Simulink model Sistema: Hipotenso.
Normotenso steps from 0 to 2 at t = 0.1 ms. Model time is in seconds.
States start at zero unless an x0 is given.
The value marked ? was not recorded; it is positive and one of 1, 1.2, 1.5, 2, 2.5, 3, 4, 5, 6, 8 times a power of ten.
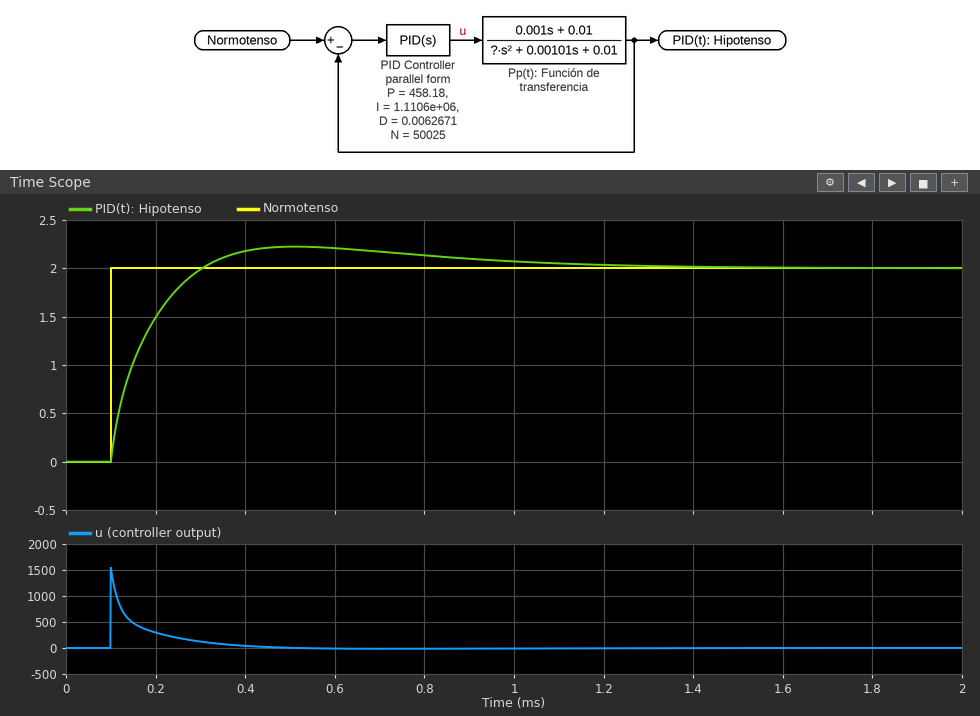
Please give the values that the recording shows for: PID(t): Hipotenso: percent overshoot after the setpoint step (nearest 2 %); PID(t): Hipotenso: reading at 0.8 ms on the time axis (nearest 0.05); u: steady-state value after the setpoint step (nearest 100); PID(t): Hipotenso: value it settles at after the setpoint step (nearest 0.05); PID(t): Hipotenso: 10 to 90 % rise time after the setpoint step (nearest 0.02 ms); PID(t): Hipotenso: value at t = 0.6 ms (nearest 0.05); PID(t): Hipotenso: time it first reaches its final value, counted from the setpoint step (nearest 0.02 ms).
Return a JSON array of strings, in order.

["12 %", "2.15", "0", "2.00", "0.14 ms", "2.20", "0.20 ms"]
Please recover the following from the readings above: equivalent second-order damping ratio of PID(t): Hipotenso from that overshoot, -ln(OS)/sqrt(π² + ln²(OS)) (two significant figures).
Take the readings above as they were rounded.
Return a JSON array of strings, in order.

["0.56"]
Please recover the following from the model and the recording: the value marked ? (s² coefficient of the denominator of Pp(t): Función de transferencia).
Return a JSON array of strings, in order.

["4e-05"]
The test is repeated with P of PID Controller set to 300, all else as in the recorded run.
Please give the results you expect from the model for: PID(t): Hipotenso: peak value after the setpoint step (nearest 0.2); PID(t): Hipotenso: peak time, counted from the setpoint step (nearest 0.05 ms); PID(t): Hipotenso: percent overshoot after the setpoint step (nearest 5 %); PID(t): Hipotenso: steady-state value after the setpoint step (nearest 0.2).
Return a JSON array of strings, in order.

["2.4", "0.45 ms", "20 %", "2.0"]
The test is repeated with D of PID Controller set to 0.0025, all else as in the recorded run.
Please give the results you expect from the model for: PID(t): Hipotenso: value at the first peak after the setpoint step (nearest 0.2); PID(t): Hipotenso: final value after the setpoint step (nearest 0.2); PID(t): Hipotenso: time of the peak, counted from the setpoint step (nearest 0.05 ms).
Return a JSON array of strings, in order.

["2.2", "2.0", "0.40 ms"]
